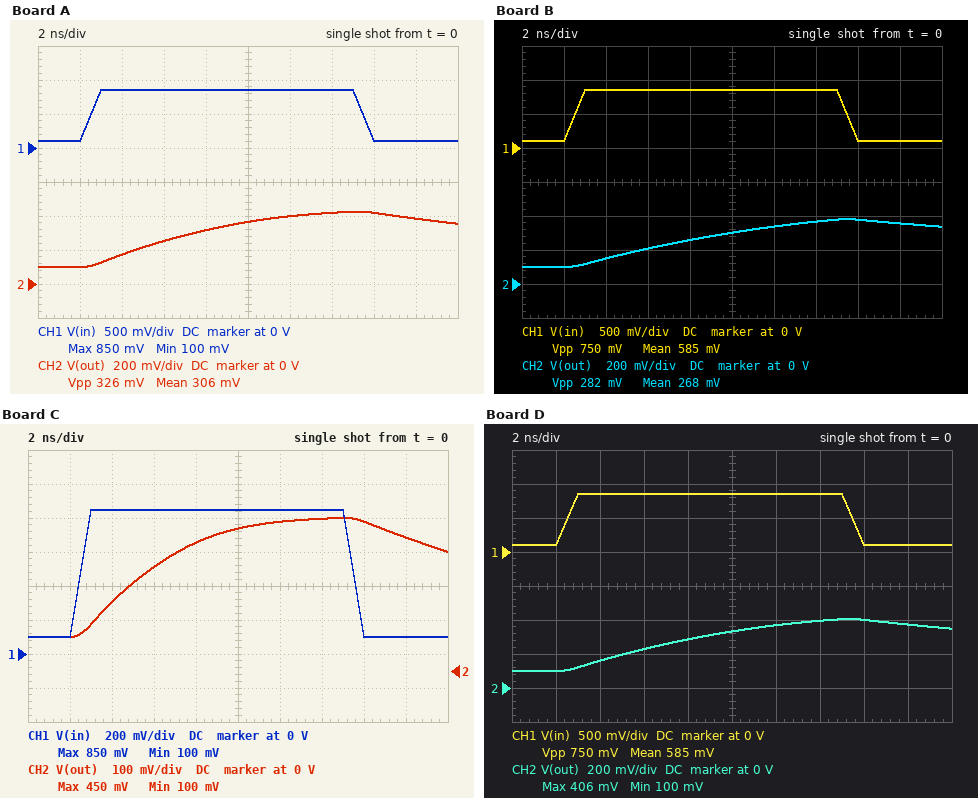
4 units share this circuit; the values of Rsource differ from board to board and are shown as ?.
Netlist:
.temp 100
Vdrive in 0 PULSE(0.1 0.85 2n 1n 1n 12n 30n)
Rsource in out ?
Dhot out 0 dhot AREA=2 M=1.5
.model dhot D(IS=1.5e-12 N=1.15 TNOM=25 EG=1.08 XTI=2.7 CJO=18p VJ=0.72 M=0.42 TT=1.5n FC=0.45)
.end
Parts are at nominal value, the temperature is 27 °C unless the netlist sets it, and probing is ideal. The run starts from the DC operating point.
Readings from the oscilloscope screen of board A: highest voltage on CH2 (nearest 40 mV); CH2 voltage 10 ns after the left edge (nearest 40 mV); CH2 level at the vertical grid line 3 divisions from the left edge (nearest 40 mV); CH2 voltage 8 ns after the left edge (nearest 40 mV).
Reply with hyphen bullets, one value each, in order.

- 440 mV
- 360 mV
- 240 mV
- 320 mV
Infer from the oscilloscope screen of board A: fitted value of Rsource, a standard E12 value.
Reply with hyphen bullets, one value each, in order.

- 220 Ω
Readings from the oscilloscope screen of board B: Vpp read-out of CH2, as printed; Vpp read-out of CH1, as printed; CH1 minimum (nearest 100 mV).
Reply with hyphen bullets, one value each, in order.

- 282 mV
- 750 mV
- 100 mV
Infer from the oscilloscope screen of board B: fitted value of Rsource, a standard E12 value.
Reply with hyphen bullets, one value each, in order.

- 330 Ω
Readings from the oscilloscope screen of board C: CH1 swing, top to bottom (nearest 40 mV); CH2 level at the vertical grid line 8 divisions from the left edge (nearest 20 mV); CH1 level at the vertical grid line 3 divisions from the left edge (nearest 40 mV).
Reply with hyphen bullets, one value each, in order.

- 760 mV
- 440 mV
- 840 mV
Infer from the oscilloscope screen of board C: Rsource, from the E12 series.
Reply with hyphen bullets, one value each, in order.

- 150 Ω
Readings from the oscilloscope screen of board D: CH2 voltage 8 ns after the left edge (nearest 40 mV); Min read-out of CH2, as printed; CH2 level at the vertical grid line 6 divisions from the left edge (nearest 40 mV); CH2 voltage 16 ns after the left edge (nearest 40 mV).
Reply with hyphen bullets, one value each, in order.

- 280 mV
- 100 mV
- 360 mV
- 400 mV
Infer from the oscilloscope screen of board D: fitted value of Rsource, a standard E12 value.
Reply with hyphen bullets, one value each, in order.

- 270 Ω
